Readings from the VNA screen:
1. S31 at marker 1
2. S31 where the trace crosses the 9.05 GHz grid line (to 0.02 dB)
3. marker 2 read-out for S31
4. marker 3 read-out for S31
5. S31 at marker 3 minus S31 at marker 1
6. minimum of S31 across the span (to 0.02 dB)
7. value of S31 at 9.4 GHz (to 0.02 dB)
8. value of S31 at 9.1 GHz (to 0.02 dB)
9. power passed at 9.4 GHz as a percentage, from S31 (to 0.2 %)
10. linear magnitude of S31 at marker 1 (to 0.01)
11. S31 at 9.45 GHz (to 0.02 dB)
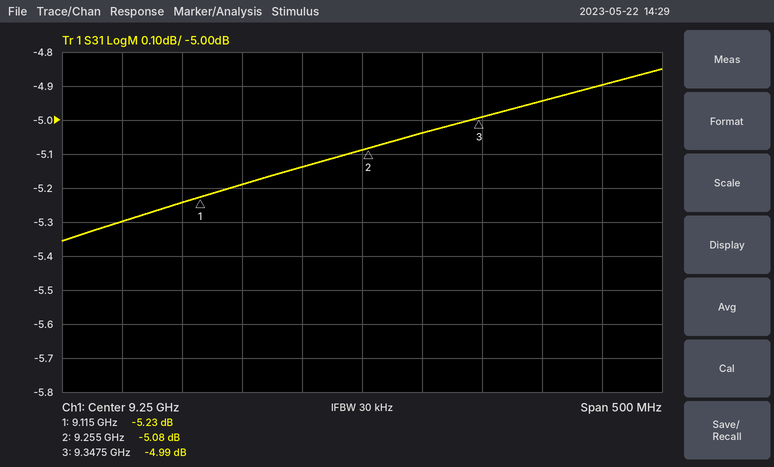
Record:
-5.23 dB
-5.30 dB
-5.08 dB
-4.99 dB
0.24 dB
-5.36 dB
-4.94 dB
-5.24 dB
32.0 %
0.55
-4.90 dB
